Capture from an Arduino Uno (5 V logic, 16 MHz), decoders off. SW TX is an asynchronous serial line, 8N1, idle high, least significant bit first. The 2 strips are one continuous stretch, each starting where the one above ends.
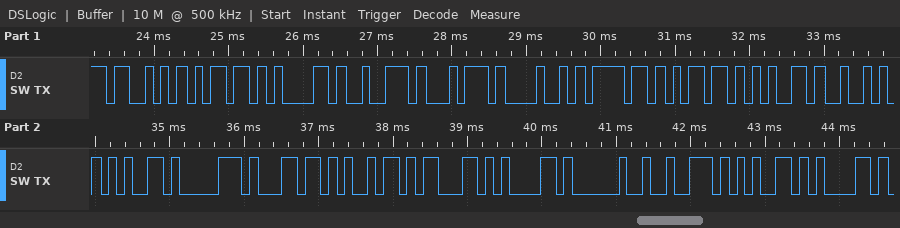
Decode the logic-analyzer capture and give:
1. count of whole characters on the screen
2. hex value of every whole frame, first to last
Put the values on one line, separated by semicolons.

20; 53 6D 61 72 74 48 6F 6D 65 52 65 70 6C 69 63 61 20 72 65 61
